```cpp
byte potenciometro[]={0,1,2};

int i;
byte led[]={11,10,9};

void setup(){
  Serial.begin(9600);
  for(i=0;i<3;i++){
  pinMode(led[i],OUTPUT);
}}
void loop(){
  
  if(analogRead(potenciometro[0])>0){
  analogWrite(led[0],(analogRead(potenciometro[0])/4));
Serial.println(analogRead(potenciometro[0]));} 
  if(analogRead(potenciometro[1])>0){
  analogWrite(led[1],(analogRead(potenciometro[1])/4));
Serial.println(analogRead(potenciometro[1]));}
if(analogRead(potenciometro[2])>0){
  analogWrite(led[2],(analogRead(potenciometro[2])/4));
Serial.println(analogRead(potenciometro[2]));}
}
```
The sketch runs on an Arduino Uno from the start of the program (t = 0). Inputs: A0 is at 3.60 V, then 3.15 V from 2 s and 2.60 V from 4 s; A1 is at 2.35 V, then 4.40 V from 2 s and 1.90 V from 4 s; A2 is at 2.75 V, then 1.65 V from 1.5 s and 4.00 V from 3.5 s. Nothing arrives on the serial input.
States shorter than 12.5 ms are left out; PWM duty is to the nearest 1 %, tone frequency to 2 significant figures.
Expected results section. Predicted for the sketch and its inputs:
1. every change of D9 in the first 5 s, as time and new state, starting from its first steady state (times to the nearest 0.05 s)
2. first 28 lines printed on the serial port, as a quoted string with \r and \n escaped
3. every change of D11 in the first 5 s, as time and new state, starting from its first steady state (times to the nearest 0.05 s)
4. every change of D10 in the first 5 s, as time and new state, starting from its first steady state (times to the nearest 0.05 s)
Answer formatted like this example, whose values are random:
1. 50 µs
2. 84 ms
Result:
1. 0 s PWM 55 %; 1.5 s PWM 33 %; 3.5 s PWM 80 %
2. "737\r\n481\r\n563\r\n737\r\n481\r\n563\r\n737\r\n481\r\n563\r\n737\r\n481\r\n563\r\n737\r\n481\r\n563\r\n737\r\n481\r\n563\r\n737\r\n481\r\n563\r\n737\r\n481\r\n563\r\n737\r\n481\r\n563\r\n737\r\n"
3. 0 s PWM 72 %; 2 s PWM 63 %; 4 s PWM 52 %
4. 0 s PWM 47 %; 2 s PWM 88 %; 4 s PWM 38 %
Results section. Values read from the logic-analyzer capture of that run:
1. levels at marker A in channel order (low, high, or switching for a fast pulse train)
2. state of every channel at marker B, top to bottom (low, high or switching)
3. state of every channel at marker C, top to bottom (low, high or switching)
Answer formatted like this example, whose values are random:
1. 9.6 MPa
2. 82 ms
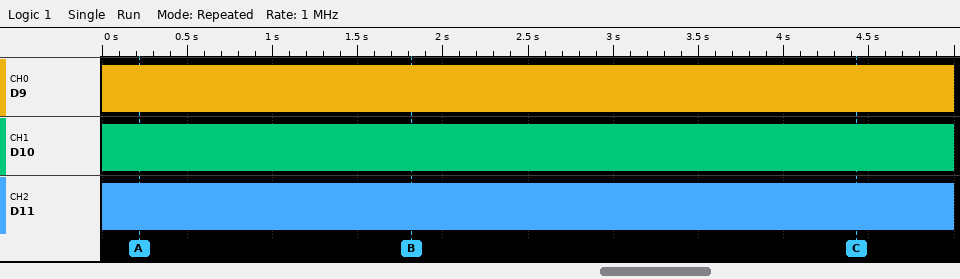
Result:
1. D9 switching, D10 switching, D11 switching
2. D9 switching, D10 switching, D11 switching
3. D9 switching, D10 switching, D11 switching
